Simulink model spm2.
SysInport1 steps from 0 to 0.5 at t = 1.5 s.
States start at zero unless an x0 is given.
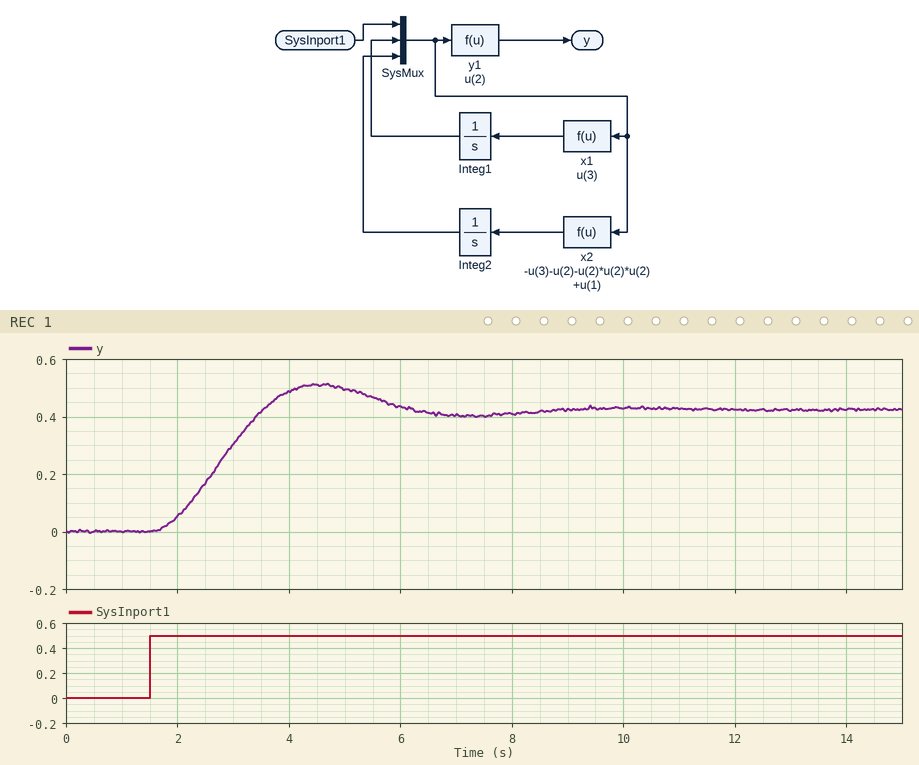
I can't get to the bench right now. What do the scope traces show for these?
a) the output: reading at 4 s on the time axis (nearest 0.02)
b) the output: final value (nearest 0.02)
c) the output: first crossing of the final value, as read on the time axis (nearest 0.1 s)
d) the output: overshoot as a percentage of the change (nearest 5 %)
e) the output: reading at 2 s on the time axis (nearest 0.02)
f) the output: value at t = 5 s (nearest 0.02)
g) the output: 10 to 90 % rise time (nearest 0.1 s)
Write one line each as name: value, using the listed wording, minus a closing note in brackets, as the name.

the output: reading at 4 s on the time axis: 0.48
the output: final value: 0.42
the output: first crossing of the final value, as read on the time axis: 3.5 s
the output: overshoot as a percentage of the change: 20 %
the output: reading at 2 s on the time axis: 0.06
the output: value at t = 5 s: 0.50
the output: 10 to 90 % rise time: 1.4 s
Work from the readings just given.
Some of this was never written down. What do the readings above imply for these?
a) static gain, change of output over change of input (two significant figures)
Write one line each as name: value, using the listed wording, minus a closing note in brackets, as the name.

static gain, change of output over change of input: 0.84
